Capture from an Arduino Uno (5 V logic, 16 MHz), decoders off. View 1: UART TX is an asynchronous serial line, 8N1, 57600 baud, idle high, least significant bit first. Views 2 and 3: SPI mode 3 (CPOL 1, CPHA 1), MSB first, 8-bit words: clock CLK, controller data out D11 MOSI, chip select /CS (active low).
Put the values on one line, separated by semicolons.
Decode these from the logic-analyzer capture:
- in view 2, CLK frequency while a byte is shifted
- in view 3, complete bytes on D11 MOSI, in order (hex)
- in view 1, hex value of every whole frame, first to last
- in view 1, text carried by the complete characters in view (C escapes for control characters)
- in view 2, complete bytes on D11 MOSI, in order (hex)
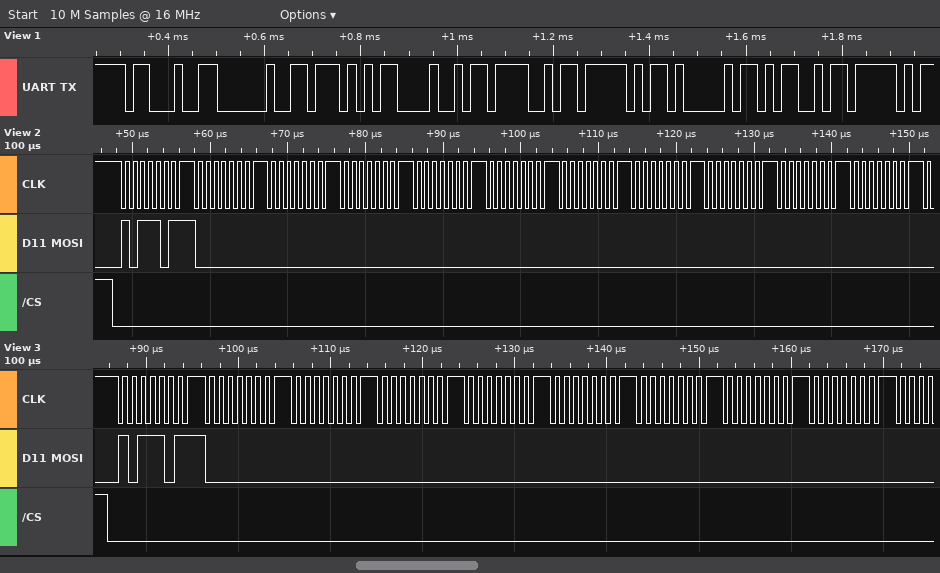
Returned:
1 MHz; BB 00 00 00 00 00 00 00 00; 23 20 57 48 4F 5F 41 4D 5F; "# WHO_AM_"; BB 00 00 00 00 00 00 00 00 00 00
